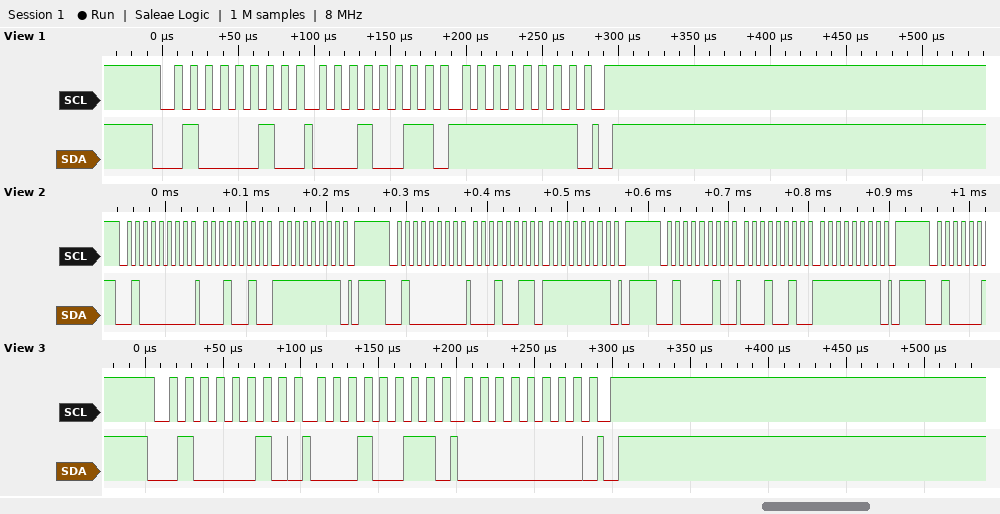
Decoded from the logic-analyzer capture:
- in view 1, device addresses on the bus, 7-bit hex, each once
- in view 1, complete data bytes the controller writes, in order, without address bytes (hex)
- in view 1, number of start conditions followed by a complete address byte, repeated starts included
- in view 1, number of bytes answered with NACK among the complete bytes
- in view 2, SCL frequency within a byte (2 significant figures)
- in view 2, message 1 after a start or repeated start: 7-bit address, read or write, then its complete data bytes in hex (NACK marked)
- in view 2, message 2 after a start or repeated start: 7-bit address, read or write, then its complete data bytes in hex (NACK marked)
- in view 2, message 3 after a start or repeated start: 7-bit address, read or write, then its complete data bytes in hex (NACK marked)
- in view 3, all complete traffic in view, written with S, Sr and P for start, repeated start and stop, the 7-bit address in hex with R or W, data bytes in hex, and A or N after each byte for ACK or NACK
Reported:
0x21
13 FF
1
0
100 kHz
0x20 write: 12 FF
0x20 write: 13 FF
0x21 write: 12 FF
S 21W A 13 A 00 A P
